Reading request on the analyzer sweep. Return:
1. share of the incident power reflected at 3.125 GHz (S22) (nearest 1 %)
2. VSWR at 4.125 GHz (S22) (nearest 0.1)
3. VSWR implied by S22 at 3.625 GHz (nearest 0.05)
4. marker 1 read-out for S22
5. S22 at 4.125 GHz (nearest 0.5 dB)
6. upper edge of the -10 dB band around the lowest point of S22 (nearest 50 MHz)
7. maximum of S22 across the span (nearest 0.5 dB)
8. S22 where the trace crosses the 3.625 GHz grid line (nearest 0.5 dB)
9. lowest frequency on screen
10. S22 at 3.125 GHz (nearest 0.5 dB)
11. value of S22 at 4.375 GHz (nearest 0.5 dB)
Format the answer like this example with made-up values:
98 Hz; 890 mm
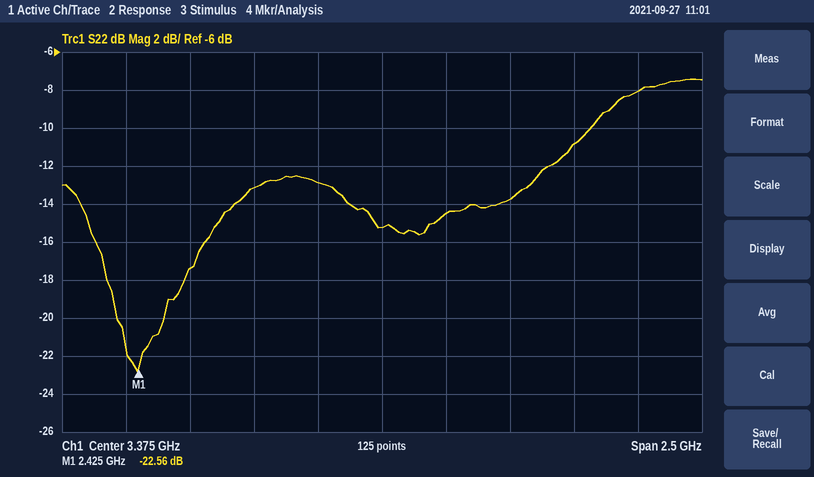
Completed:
5 %; 1.8; 1.45; -22.56 dB; -11.0 dB; 4.20 GHz; -7.5 dB; -14.5 dB; 2.125 GHz; -13.0 dB; -8.0 dB
